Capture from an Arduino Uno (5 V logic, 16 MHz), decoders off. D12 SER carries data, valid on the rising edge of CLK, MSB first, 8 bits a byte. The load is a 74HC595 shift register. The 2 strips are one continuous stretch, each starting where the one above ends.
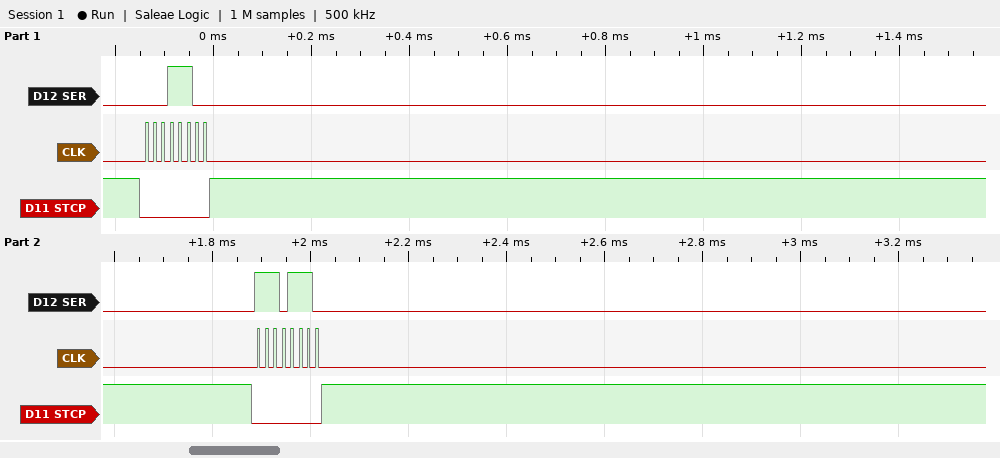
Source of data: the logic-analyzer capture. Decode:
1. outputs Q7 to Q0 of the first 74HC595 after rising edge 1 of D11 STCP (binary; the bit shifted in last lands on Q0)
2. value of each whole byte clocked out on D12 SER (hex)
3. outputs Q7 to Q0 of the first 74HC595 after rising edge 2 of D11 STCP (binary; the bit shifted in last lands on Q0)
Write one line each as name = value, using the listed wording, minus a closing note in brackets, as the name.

outputs Q7 to Q0 of the first 74HC595 after rising edge 1 of D11 STCP = 00011100
value of each whole byte clocked out on D12 SER = 1C EE
outputs Q7 to Q0 of the first 74HC595 after rising edge 2 of D11 STCP = 11101110
